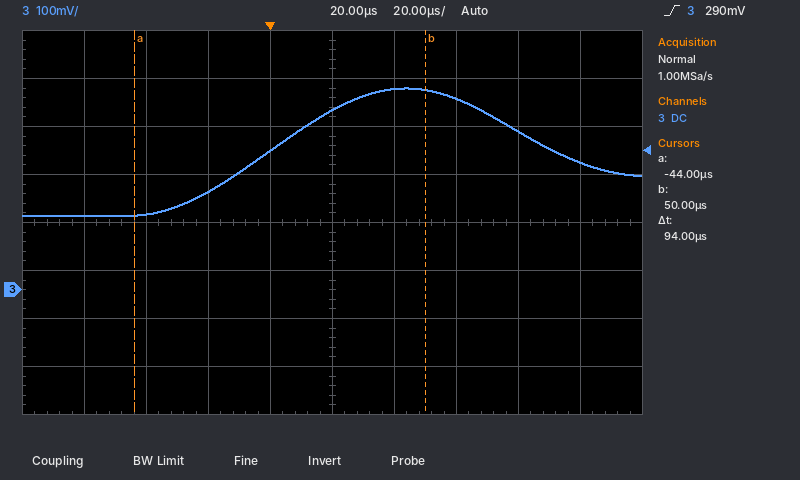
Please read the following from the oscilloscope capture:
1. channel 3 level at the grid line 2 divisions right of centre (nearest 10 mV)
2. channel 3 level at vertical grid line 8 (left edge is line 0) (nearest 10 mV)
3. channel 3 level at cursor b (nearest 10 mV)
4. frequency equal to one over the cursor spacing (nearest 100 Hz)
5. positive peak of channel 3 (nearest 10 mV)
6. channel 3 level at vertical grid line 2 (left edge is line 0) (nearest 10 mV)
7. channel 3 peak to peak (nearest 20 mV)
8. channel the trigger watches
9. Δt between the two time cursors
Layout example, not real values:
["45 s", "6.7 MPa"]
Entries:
["400 mV", "330 mV", "420 mV", "10.6 kHz", "420 mV", "160 mV", "260 mV", "channel 3", "94 µs"]
